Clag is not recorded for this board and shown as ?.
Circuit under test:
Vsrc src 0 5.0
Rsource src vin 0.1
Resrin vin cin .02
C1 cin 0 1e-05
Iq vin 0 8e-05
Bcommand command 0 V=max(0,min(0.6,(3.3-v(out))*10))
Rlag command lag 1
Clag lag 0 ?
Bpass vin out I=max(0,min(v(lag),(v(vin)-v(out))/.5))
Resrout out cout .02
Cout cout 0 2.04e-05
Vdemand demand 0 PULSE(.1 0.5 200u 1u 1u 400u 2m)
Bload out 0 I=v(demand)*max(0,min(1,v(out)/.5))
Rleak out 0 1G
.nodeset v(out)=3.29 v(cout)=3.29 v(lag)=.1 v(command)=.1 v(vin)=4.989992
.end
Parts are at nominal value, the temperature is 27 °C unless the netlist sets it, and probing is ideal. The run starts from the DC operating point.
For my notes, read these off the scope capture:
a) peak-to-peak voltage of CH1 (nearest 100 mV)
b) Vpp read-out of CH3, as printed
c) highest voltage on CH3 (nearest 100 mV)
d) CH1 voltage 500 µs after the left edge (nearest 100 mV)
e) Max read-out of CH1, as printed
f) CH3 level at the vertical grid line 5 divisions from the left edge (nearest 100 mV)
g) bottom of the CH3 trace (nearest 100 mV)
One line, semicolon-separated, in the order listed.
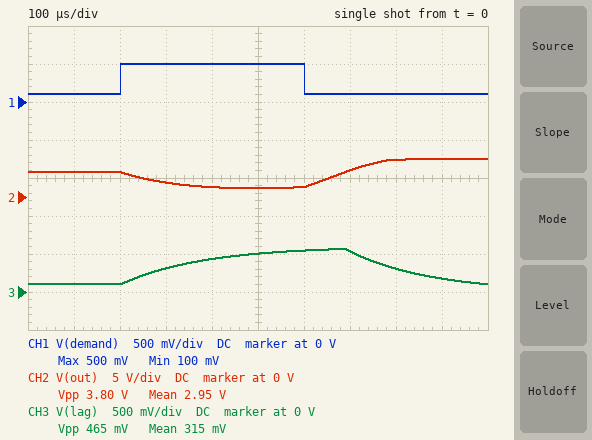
400 mV; 465 mV; 600 mV; 500 mV; 500 mV; 500 mV; 100 mV
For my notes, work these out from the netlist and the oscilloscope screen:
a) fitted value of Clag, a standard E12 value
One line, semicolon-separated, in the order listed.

180 µF
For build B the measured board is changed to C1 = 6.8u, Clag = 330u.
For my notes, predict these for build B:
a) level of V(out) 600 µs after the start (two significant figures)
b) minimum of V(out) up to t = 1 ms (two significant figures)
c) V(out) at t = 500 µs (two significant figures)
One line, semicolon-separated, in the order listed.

440 mV; 370 mV; 390 mV
